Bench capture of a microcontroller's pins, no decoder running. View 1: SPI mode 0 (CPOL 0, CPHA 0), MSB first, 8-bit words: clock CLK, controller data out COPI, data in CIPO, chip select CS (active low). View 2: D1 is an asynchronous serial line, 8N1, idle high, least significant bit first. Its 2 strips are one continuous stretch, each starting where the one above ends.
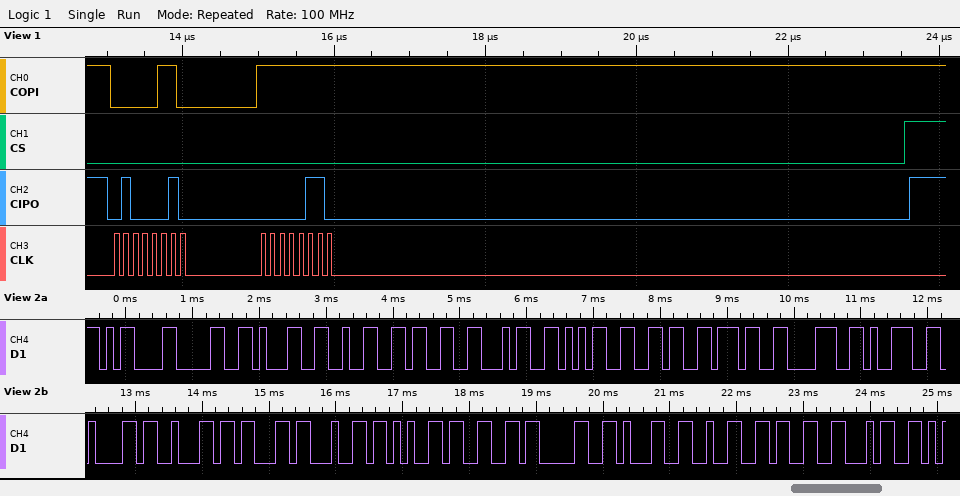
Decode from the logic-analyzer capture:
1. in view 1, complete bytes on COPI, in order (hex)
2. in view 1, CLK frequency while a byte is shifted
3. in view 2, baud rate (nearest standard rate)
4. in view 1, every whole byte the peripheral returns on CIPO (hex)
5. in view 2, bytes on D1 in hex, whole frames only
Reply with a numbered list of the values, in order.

1. 06 FF
2. 8 MHz
3. 9600 baud
4. 42 06
5. 0D 30 31 32 33 34 35 36 37 38 39 61 62 63 64 65 66 30 31 32 33 34
